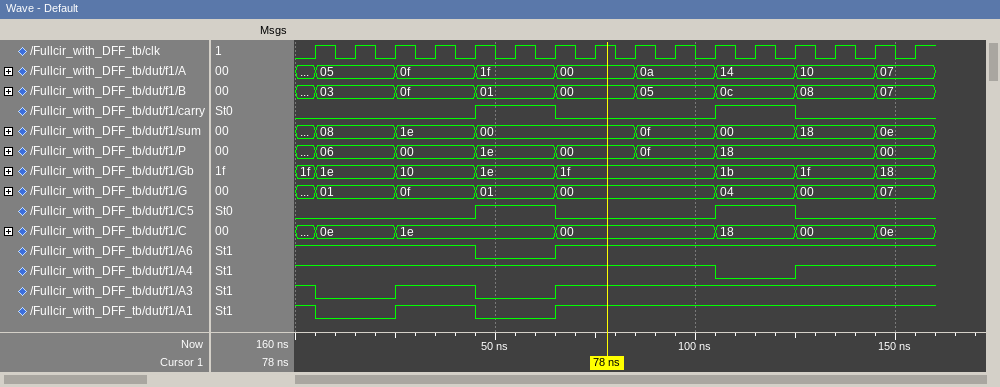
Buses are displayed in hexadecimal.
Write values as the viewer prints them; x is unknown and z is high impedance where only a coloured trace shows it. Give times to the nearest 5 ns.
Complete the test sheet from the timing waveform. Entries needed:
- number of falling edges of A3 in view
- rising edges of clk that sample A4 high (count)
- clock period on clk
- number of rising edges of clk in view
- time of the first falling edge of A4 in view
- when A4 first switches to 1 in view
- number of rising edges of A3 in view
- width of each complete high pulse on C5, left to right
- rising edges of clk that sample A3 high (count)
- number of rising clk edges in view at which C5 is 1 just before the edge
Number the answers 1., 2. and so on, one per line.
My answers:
1. 2
2. 14
3. 10 ns
4. 16
5. 105 ns
6. 125 ns
7. 2
8. 20 ns, 20 ns
9. 12
10. 4
